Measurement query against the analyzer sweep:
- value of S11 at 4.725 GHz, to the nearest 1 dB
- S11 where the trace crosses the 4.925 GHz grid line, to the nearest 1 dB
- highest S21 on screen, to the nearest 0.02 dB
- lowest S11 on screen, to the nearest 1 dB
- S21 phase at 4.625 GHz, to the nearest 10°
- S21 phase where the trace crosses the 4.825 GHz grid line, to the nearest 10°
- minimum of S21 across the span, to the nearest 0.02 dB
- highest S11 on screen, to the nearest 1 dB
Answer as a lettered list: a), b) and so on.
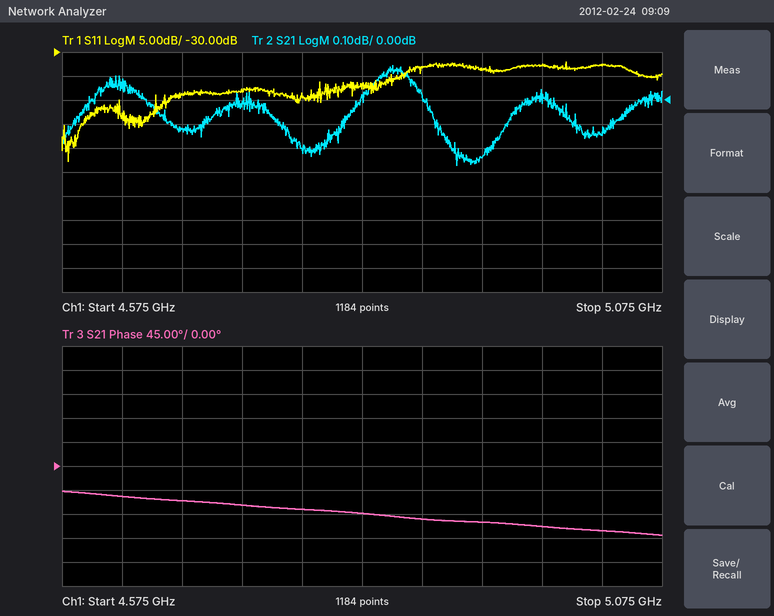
a) -38 dB
b) -34 dB
c) 0.14 dB
d) -53 dB
e) -60°
f) -90°
g) -0.28 dB
h) -32 dB
